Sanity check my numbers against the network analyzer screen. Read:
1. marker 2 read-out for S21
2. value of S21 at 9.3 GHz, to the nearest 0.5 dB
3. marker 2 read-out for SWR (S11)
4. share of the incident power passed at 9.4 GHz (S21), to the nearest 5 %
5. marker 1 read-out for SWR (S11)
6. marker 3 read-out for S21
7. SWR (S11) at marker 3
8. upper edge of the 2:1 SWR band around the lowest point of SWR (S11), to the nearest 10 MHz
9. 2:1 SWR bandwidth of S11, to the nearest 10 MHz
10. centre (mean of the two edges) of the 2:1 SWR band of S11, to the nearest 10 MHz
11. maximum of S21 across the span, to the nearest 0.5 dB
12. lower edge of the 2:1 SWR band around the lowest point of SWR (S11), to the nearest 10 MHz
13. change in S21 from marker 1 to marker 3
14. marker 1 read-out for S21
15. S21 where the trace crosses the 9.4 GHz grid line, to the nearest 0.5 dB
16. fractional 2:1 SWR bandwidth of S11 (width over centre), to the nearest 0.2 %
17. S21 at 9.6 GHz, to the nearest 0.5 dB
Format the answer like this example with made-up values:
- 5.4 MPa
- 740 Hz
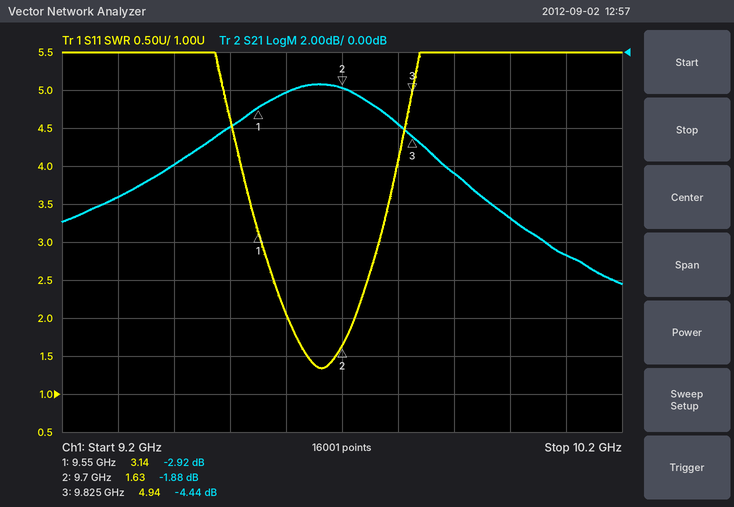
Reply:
- -1.88 dB
- -7.5 dB
- 1.63
- 25 %
- 3.14
- -4.44 dB
- 4.94
- 9.72 GHz
- 120 MHz
- 9.66 GHz
- -1.5 dB
- 9.60 GHz
- -1.52 dB
- -2.92 dB
- -6.0 dB
- 1.2 %
- -2.0 dB
